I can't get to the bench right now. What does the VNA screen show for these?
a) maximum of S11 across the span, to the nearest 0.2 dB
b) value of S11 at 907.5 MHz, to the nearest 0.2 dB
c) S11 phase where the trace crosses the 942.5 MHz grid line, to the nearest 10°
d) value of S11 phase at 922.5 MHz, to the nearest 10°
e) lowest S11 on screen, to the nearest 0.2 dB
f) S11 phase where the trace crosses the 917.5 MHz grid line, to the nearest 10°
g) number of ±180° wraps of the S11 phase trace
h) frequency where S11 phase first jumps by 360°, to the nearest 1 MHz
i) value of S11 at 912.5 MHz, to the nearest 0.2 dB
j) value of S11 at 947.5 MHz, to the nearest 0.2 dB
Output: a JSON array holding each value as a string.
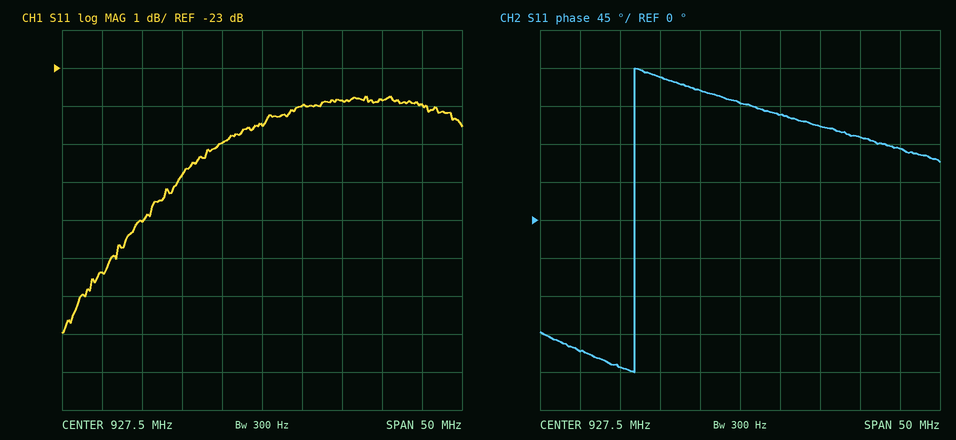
["-23.8 dB", "-28.4 dB", "100°", "150°", "-30.0 dB", "170°", "1", "914 MHz", "-27.0 dB", "-24.0 dB"]
